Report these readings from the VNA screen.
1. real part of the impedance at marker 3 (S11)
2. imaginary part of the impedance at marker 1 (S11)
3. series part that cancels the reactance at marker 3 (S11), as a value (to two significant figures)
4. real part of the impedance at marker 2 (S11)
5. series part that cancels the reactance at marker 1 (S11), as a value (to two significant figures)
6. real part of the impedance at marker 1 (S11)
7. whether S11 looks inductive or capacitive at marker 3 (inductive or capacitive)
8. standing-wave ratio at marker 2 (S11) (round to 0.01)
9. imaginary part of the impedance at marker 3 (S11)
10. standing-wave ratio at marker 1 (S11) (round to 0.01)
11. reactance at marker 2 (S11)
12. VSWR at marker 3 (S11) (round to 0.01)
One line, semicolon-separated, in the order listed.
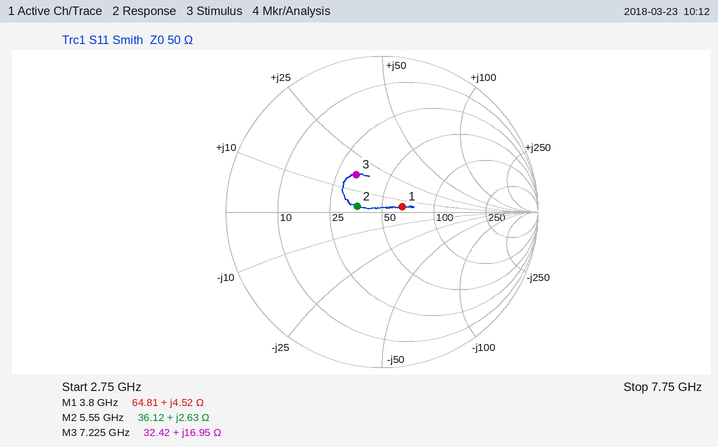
32.42 Ω; +4.52 Ω; 1.3 pF; 36.12 Ω; 9.3 pF; 64.81 Ω; inductive; 1.39; +16.95 Ω; 1.31; +2.63 Ω; 1.82
